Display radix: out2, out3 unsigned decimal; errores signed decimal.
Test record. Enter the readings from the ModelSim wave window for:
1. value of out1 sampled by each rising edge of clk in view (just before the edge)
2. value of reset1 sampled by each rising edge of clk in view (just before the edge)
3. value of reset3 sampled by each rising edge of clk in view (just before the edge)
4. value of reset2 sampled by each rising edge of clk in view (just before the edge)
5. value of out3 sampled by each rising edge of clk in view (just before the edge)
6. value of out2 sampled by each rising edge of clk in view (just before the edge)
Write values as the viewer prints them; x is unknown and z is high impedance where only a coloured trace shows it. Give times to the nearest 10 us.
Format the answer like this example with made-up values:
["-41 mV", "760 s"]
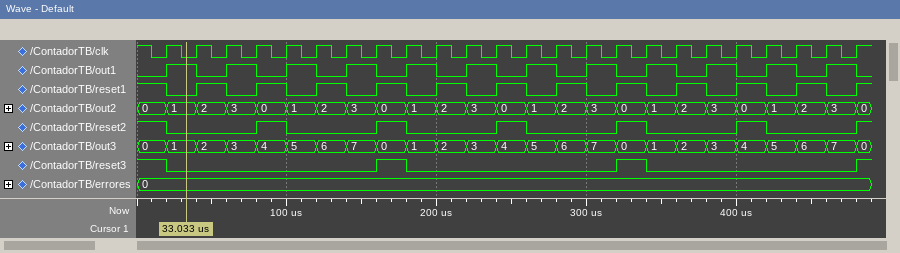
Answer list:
["0 1 0 1 0 1 0 1 0 1 0 1 0 1 0 1 0 1 0 1 0 1 0 1", "1 0 1 0 1 0 1 0 1 0 1 0 1 0 1 0 1 0 1 0 1 0 1 0", "1 0 0 0 0 0 0 0 1 0 0 0 0 0 0 0 1 0 0 0 0 0 0 0", "1 0 0 0 1 0 0 0 1 0 0 0 1 0 0 0 1 0 0 0 1 0 0 0", "0, 1, 2, 3, 4, 5, 6, 7, 0, 1, 2, 3, 4, 5, 6, 7, 0, 1, 2, 3, 4, 5, 6, 7", "0, 1, 2, 3, 0, 1, 2, 3, 0, 1, 2, 3, 0, 1, 2, 3, 0, 1, 2, 3, 0, 1, 2, 3"]
